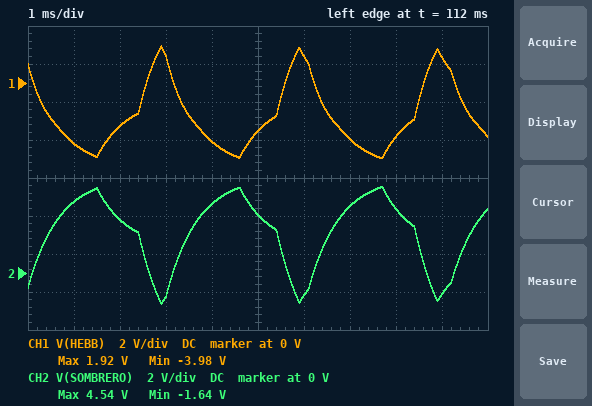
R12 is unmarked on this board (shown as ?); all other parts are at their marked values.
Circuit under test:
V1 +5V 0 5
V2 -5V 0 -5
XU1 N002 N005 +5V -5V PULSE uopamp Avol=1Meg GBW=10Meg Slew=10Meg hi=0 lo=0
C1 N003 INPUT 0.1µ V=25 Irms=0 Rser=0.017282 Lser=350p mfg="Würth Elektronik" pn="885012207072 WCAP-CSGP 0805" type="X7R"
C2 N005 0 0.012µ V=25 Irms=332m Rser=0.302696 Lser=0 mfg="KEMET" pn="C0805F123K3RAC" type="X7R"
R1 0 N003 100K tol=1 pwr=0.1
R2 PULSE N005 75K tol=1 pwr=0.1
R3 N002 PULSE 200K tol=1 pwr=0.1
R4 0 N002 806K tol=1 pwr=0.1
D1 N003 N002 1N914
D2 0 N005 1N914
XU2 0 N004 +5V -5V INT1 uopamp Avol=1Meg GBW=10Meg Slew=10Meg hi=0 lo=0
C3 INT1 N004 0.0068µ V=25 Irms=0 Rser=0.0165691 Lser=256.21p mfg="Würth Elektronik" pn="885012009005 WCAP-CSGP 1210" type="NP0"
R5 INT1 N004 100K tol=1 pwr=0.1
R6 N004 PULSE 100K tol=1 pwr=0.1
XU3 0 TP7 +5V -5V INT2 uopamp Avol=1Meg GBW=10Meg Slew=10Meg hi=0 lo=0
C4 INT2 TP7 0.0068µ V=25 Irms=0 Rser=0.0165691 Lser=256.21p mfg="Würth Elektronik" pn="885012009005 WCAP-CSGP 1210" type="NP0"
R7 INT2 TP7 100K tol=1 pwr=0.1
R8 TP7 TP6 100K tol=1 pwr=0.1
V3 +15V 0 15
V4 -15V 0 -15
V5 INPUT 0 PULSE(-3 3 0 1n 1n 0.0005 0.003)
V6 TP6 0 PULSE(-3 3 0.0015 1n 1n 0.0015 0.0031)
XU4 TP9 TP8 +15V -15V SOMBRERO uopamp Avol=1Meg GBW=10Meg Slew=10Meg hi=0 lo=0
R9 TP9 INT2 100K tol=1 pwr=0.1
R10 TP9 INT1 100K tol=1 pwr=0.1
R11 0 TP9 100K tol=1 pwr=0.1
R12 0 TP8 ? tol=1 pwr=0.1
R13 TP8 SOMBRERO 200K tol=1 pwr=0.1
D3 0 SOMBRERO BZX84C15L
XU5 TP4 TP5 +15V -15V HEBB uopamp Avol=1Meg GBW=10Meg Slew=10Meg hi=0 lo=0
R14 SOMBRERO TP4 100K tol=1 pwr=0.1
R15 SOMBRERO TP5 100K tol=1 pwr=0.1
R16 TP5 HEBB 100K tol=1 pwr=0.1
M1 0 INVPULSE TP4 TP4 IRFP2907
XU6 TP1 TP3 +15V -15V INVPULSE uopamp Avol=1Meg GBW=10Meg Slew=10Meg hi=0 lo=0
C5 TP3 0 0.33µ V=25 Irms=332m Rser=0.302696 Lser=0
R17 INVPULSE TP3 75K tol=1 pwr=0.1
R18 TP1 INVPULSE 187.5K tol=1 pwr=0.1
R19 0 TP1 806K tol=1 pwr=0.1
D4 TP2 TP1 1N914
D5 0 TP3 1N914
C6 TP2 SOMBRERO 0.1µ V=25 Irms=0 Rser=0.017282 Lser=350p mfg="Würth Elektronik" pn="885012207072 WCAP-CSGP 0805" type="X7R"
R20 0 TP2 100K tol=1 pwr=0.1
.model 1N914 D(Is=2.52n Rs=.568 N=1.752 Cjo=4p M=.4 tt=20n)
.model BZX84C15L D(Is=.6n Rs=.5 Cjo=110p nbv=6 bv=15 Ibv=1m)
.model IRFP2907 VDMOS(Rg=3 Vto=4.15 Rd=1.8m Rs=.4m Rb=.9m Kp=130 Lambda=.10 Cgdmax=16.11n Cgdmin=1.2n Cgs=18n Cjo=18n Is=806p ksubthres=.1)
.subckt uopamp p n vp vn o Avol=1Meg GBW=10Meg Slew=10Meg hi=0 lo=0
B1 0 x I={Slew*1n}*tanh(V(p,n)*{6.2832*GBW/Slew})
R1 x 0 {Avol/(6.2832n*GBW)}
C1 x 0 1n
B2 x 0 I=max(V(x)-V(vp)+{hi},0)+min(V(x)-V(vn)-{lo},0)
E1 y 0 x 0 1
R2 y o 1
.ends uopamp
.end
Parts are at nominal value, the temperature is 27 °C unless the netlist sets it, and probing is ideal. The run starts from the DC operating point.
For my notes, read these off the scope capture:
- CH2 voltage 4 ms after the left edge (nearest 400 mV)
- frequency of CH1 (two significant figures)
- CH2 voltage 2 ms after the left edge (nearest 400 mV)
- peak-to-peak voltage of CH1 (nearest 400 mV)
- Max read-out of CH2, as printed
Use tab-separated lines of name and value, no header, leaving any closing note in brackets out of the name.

CH2 voltage 4 ms after the left edge	3.6 V
frequency of CH1	330 Hz
CH2 voltage 2 ms after the left edge	2.8 V
peak-to-peak voltage of CH1	6.0 V
Max read-out of CH2, as printed	4.54 V
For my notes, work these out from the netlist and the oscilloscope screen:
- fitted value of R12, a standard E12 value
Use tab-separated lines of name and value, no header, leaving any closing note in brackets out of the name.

fitted value of R12, a standard E12 value	220 kΩ
